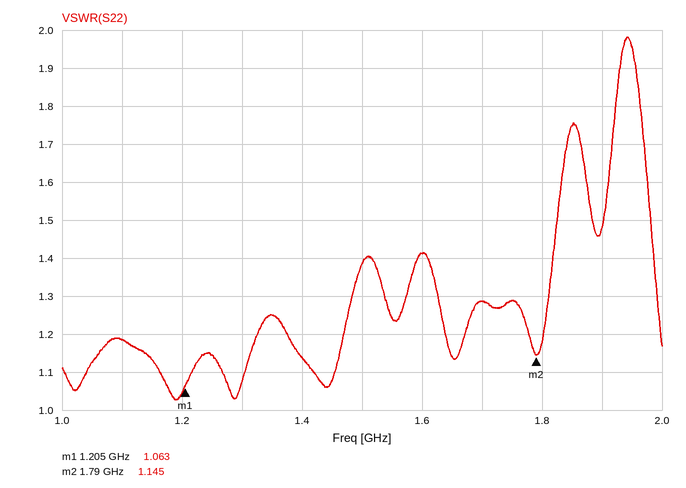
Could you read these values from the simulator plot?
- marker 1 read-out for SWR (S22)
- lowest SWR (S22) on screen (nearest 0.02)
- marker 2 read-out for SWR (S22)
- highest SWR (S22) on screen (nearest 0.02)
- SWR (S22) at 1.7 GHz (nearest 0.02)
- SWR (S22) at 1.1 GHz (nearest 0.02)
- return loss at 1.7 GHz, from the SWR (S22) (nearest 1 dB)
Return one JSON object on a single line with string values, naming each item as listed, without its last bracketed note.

{"marker 1 read-out for SWR": "1.063", "lowest SWR (S22) on screen": "1.02", "marker 2 read-out for SWR": "1.145", "highest SWR (S22) on screen": "1.98", "SWR (S22) at 1.7 GHz": "1.28", "SWR (S22) at 1.1 GHz": "1.18", "return loss at 1.7 GHz, from the SWR (S22)": "18 dB"}
